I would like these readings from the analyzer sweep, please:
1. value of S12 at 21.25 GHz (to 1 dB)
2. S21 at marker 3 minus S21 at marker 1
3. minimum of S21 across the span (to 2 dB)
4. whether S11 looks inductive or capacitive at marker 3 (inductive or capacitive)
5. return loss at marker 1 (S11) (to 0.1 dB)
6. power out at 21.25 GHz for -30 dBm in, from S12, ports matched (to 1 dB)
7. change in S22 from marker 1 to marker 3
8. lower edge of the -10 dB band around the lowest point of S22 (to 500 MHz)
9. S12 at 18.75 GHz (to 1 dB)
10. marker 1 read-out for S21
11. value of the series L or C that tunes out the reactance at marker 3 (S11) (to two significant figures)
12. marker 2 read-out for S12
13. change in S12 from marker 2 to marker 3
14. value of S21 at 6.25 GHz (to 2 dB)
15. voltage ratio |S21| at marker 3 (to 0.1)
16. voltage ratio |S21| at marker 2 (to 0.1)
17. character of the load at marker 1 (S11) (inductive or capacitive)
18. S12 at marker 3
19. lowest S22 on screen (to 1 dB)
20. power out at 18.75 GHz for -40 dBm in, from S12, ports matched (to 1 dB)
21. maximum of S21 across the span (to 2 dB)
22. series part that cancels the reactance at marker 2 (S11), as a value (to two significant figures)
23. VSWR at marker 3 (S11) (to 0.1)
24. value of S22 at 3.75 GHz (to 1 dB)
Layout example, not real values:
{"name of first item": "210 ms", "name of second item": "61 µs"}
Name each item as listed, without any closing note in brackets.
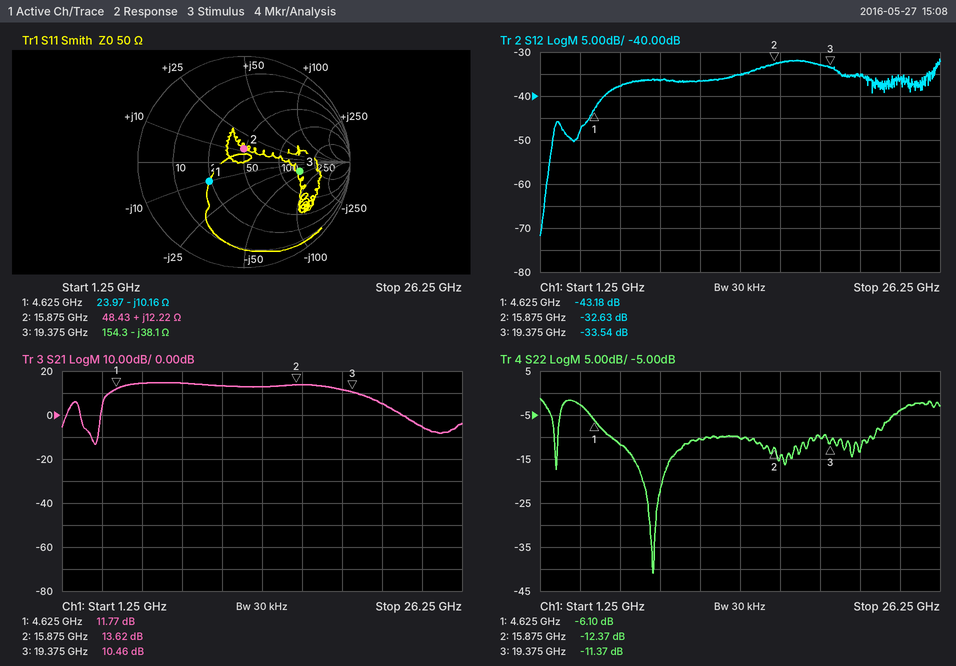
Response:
{"value of S12 at 21.25 GHz": "-35 dB", "S21 at marker 3 minus S21 at marker 1": "-1.31 dB", "minimum of S21 across the span": "-14 dB", "whether S11 looks inductive or capacitive at marker 3": "capacitive", "return loss at marker 1 (S11)": "8.5 dB", "power out at 21.25 GHz for -30 dBm in, from S12, ports matched": "-65 dBm", "change in S22 from marker 1 to marker 3": "-5.27 dB", "lower edge of the -10 dB band around the lowest point of S22": "5.5 GHz", "S12 at 18.75 GHz": "-33 dB", "marker 1 read-out for S21": "11.77 dB", "value of the series L or C that tunes out the reactance at marker 3 (S11)": "310 pH", "marker 2 read-out for S12": "-32.63 dB", "change in S12 from marker 2 to marker 3": "-0.91 dB", "value of S21 at 6.25 GHz": "14 dB", "voltage ratio |S21| at marker 3": "3.3", "voltage ratio |S21| at marker 2": "4.8", "character of the load at marker 1 (S11)": "capacitive", "S12 at marker 3": "-33.54 dB", "lowest S22 on screen": "-41 dB", "power out at 18.75 GHz for -40 dBm in, from S12, ports matched": "-73 dBm", "maximum of S21 across the span": "14 dB", "series part that cancels the reactance at marker 2 (S11), as a value": "820 fF", "VSWR at marker 3 (S11)": "3.3", "value of S22 at 3.75 GHz": "-3 dB"}
